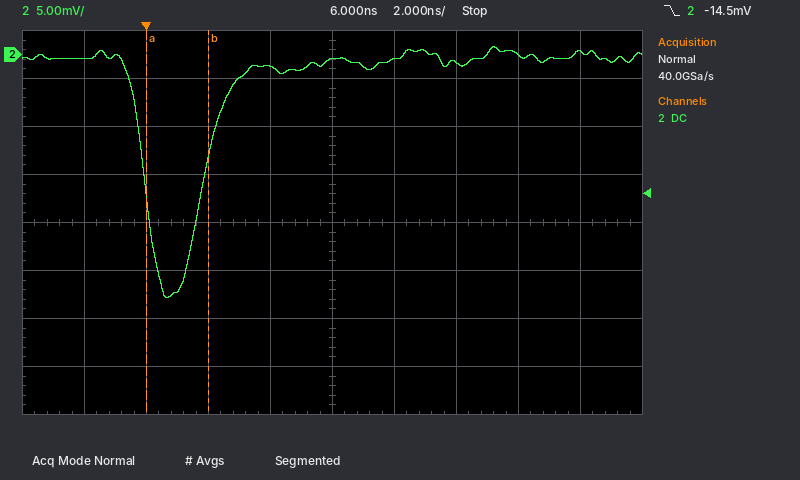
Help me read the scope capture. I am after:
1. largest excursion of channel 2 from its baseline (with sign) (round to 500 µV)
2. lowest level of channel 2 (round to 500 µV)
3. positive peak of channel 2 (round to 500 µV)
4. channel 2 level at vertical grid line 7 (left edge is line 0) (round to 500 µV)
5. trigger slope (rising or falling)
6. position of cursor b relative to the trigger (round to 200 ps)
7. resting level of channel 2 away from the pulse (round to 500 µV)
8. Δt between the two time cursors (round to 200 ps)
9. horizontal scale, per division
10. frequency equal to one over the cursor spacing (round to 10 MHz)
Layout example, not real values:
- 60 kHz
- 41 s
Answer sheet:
- -25.0 mV
- -25.5 mV
- 1.0 mV
- -1.0 mV
- falling
- +2.0 ns
- -500 µV
- 2.0 ns
- 2 ns
- 500 MHz
